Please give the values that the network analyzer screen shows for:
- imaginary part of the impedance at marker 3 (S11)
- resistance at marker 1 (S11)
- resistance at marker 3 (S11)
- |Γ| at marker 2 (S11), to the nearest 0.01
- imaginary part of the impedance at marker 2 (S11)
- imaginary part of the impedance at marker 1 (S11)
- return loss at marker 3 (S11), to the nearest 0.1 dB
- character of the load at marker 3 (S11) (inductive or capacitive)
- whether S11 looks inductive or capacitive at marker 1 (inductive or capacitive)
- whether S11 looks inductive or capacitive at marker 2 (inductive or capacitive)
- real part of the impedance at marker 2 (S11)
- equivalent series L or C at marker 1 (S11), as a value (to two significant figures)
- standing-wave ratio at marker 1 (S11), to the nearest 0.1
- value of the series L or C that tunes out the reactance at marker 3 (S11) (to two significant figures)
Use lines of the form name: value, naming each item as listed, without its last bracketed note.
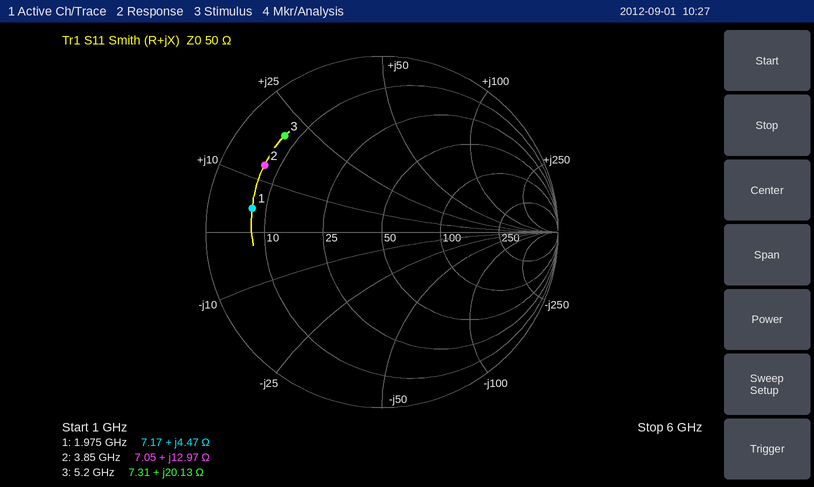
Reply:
imaginary part of the impedance at marker 3: +20.13 Ω
resistance at marker 1: 7.17 Ω
resistance at marker 3: 7.31 Ω
|Γ| at marker 2 (S11), to the nearest 0.01: 0.77
imaginary part of the impedance at marker 2: +12.97 Ω
imaginary part of the impedance at marker 1: +4.47 Ω
return loss at marker 3 (S11), to the nearest 0.1 dB: 2.2 dB
character of the load at marker 3 (S11): inductive
whether S11 looks inductive or capacitive at marker 1: inductive
whether S11 looks inductive or capacitive at marker 2: inductive
real part of the impedance at marker 2: 7.05 Ω
equivalent series L or C at marker 1 (S11), as a value: 360 pH
standing-wave ratio at marker 1 (S11), to the nearest 0.1: 7.0
value of the series L or C that tunes out the reactance at marker 3 (S11): 1.5 pF
